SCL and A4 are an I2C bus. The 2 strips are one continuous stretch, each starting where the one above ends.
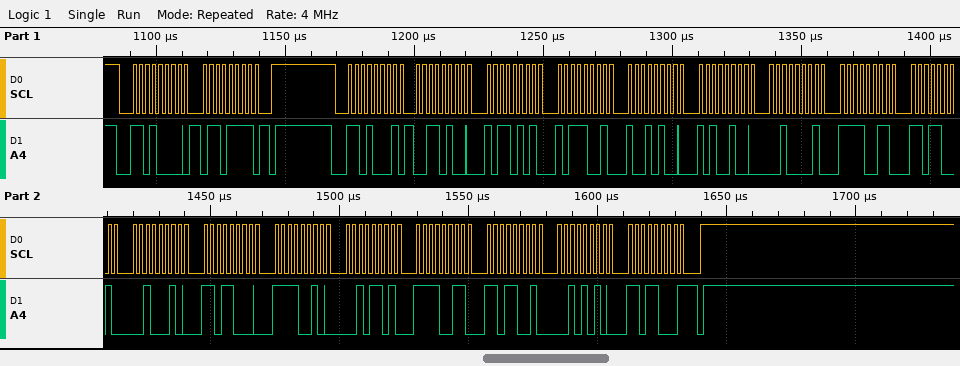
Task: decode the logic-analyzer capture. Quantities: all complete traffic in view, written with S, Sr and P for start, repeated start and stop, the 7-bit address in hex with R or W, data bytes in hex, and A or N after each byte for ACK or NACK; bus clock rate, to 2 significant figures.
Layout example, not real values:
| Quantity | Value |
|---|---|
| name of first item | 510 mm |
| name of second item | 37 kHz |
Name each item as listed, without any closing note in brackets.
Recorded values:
| Quantity | Value |
|---|---|
| all complete traffic in view, written with S, Sr and P for start, repeated start and stop, the 7-bit address in hex with R or W, data bytes in hex, and A or N after each byte for ACK or NACK | S 68W A 6F A P S 68R A 34 A B5 A B9 A 94 A A4 A 21 A F3 A D9 A 22 A D8 A F2 A 2D A F3 A D9 A 2A A D8 N P |
| bus clock rate, to 2 significant figures | 400 kHz |
